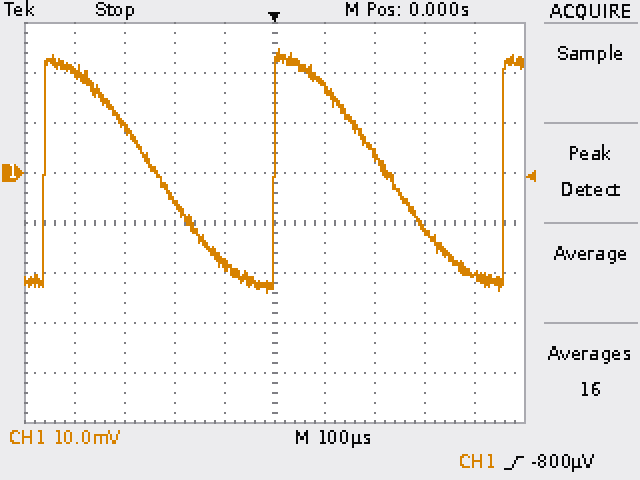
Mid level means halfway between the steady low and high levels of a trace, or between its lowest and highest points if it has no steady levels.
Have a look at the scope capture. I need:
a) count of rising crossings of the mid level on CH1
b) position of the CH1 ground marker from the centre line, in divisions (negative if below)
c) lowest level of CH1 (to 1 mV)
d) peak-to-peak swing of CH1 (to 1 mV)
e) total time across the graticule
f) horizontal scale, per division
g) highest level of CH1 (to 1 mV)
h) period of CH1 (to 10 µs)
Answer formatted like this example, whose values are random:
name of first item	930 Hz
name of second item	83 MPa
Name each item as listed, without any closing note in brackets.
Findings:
count of rising crossings of the mid level on CH1	3
position of the CH1 ground marker from the centre line, in divisions	+1.0 div
lowest level of CH1	-24 mV
peak-to-peak swing of CH1	49 mV
total time across the graticule	1 ms
horizontal scale, per division	100 µs
highest level of CH1	25 mV
period of CH1	460 µs
